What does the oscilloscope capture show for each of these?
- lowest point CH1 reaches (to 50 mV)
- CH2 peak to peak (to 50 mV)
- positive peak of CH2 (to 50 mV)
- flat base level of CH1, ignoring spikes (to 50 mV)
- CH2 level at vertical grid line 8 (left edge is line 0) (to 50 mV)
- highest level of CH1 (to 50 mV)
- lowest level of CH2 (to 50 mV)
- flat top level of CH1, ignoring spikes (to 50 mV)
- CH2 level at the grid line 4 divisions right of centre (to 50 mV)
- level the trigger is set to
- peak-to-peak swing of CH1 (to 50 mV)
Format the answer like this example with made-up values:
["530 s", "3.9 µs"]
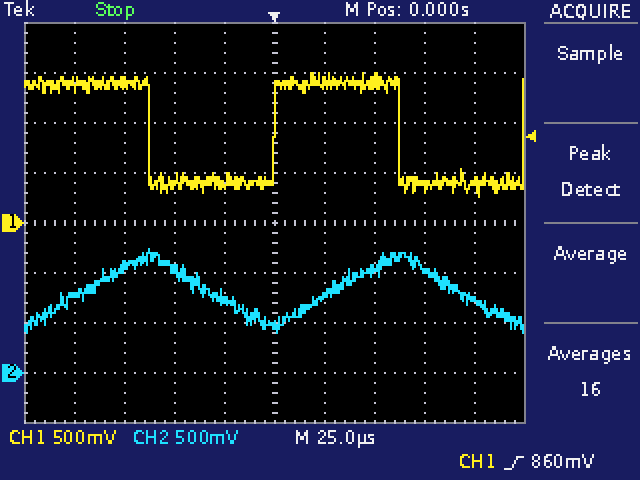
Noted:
["250 mV", "850 mV", "1.25 V", "400 mV", "1.05 V", "1.50 V", "400 mV", "1.40 V", "700 mV", "860 mV", "1.25 V"]
